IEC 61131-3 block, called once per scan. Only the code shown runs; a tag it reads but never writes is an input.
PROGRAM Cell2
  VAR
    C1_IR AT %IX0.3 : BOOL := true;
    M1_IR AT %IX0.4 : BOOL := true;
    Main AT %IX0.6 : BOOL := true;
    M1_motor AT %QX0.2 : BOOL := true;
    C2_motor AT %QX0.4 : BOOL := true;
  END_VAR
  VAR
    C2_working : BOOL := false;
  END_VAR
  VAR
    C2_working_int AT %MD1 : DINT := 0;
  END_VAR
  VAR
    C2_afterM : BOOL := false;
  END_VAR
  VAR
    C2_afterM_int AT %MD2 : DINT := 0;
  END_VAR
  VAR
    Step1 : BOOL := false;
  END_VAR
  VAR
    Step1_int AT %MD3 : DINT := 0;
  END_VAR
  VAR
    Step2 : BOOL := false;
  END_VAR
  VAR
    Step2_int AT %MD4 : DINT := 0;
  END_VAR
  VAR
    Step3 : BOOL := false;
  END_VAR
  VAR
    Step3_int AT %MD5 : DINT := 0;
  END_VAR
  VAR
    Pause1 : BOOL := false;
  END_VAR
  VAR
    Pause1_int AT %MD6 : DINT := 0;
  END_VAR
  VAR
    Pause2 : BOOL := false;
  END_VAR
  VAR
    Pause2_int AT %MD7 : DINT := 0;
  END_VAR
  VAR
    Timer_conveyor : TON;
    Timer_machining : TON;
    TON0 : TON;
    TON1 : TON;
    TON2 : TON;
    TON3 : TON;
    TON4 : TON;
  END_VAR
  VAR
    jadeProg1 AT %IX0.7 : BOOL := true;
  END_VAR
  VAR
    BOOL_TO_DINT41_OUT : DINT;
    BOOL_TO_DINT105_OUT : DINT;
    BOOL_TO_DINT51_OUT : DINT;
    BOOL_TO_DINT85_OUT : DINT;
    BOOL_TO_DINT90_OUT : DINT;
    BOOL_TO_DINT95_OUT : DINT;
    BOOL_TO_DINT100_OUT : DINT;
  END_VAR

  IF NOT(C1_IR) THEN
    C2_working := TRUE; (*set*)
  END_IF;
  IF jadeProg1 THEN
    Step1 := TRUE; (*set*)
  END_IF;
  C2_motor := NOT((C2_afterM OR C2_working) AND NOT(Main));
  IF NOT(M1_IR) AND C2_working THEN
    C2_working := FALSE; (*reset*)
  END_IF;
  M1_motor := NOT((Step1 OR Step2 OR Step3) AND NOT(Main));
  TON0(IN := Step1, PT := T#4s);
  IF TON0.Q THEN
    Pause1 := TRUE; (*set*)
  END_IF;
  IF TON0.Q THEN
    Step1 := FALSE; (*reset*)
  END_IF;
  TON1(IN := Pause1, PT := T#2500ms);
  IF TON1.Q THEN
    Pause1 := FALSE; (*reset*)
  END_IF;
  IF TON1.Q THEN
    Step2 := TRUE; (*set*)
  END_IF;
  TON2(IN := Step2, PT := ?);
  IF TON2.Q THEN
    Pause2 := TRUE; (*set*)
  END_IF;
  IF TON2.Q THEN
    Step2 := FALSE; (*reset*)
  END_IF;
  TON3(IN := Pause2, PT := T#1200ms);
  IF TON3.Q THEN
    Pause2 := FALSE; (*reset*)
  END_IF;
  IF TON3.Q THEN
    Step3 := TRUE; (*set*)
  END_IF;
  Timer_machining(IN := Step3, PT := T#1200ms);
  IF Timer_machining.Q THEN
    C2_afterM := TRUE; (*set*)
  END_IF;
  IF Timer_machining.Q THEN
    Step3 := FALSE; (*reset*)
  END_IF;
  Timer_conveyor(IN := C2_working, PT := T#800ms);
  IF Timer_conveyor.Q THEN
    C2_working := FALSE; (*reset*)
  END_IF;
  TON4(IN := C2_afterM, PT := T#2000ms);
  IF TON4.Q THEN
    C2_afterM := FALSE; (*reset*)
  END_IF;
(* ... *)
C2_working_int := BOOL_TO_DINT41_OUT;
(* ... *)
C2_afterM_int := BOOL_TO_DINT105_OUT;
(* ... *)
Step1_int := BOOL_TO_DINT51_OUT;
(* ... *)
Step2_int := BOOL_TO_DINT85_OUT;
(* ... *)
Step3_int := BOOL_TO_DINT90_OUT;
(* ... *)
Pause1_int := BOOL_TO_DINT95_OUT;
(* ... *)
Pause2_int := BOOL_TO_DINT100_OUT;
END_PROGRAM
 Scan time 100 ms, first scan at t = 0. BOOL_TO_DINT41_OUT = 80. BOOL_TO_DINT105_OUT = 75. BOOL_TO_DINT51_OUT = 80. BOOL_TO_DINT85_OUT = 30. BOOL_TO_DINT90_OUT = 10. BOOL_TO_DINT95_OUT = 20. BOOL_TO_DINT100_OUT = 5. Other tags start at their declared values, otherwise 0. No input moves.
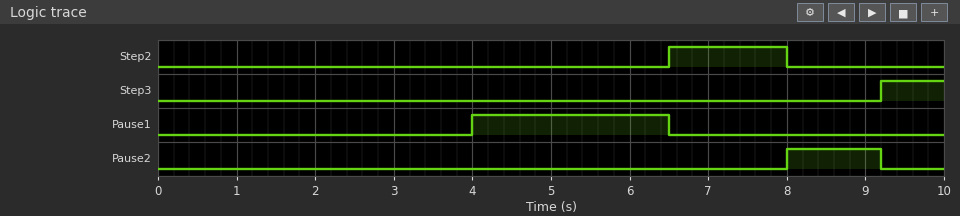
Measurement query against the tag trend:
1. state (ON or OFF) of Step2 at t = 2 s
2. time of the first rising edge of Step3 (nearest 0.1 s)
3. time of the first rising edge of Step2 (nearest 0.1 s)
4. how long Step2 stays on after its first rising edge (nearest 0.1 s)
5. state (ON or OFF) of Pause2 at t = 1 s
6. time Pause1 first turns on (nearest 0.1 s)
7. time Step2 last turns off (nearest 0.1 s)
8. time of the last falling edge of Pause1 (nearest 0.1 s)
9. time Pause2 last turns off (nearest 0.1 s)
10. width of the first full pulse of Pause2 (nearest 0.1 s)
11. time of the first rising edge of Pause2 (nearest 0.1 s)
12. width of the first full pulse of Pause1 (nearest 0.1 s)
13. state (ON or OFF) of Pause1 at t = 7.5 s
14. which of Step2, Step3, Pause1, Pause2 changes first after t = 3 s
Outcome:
OFF
9.2 s
6.5 s
1.5 s
OFF
4.0 s
8.0 s
6.5 s
9.2 s
1.2 s
8.0 s
2.5 s
OFF
Pause1
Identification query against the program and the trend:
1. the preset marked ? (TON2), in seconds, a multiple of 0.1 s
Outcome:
1.5 s
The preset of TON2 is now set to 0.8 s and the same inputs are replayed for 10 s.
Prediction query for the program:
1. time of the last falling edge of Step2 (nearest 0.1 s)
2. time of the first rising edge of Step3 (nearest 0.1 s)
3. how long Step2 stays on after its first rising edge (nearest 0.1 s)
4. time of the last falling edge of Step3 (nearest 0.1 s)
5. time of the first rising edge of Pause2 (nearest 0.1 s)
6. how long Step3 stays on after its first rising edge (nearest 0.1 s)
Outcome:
7.3 s
8.5 s
0.8 s
9.7 s
7.3 s
1.2 s
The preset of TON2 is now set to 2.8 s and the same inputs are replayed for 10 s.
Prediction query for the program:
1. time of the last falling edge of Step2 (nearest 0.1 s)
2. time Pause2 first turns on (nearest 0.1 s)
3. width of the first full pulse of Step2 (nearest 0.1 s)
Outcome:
9.3 s
9.3 s
2.8 s
